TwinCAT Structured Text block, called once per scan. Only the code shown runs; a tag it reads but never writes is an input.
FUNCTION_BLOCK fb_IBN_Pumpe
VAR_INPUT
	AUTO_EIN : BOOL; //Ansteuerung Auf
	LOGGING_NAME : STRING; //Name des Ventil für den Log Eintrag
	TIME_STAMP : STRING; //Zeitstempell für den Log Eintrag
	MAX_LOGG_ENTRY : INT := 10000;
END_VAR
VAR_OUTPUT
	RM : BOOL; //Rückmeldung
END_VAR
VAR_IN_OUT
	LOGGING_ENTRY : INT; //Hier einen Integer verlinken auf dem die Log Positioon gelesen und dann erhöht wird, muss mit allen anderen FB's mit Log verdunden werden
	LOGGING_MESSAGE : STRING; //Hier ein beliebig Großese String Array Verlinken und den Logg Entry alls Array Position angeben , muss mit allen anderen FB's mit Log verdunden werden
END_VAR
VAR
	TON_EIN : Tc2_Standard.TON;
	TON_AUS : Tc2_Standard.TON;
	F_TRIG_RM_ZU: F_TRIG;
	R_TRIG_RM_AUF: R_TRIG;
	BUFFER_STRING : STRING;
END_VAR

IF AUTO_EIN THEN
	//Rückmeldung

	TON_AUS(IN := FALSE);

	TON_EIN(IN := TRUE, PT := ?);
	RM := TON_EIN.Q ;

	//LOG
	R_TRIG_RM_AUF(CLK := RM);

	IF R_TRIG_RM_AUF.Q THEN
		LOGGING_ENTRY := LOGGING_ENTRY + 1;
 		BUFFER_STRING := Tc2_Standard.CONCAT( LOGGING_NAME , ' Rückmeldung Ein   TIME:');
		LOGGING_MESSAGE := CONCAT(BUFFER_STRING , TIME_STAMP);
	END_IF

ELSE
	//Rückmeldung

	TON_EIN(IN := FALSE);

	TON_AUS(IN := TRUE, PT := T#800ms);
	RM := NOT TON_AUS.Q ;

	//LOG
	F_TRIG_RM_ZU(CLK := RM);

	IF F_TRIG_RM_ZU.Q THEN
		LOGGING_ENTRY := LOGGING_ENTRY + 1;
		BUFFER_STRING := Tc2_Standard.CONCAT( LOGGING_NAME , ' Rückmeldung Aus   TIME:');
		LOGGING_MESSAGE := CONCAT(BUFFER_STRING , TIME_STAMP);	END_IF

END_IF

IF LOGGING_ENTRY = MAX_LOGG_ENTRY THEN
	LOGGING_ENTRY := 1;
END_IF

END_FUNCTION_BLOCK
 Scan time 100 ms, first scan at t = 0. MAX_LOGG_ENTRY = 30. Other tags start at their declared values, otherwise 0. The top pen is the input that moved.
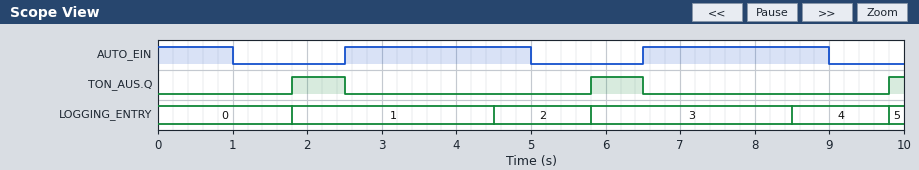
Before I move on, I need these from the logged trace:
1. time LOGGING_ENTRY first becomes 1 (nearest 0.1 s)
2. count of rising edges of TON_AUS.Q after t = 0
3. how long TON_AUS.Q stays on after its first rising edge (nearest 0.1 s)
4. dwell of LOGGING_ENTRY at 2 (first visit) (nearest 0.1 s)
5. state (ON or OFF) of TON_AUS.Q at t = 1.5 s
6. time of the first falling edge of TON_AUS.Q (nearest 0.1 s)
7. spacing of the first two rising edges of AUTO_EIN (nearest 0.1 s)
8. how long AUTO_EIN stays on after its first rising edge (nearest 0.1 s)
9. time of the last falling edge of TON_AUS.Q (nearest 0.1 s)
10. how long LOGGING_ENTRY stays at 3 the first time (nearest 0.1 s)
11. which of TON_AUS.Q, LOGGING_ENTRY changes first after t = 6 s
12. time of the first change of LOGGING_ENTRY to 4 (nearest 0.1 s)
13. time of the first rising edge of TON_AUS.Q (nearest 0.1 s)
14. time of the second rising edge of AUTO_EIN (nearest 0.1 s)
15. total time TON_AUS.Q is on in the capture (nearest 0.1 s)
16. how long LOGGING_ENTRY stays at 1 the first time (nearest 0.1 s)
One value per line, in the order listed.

1.8 s
3
0.7 s
1.3 s
OFF
2.5 s
4.0 s
2.5 s
6.5 s
2.7 s
TON_AUS.Q
8.5 s
1.8 s
6.5 s
1.6 s
2.7 s
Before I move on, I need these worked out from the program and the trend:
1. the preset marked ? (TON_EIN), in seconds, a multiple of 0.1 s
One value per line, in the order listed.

2.0 s
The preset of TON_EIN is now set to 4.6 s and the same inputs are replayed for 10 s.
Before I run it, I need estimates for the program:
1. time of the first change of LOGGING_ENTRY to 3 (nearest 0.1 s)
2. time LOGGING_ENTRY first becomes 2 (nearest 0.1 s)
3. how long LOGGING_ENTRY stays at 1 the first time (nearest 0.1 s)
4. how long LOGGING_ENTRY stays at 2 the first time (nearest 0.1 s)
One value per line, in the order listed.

9.8 s
5.8 s
4.0 s
4.0 s
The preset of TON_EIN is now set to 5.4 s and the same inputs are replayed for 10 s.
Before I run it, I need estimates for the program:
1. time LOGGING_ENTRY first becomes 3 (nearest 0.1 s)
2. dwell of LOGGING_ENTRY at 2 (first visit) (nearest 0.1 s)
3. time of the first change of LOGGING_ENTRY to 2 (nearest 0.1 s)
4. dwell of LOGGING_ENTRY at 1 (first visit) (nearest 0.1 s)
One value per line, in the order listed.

9.8 s
4.0 s
5.8 s
4.0 s
